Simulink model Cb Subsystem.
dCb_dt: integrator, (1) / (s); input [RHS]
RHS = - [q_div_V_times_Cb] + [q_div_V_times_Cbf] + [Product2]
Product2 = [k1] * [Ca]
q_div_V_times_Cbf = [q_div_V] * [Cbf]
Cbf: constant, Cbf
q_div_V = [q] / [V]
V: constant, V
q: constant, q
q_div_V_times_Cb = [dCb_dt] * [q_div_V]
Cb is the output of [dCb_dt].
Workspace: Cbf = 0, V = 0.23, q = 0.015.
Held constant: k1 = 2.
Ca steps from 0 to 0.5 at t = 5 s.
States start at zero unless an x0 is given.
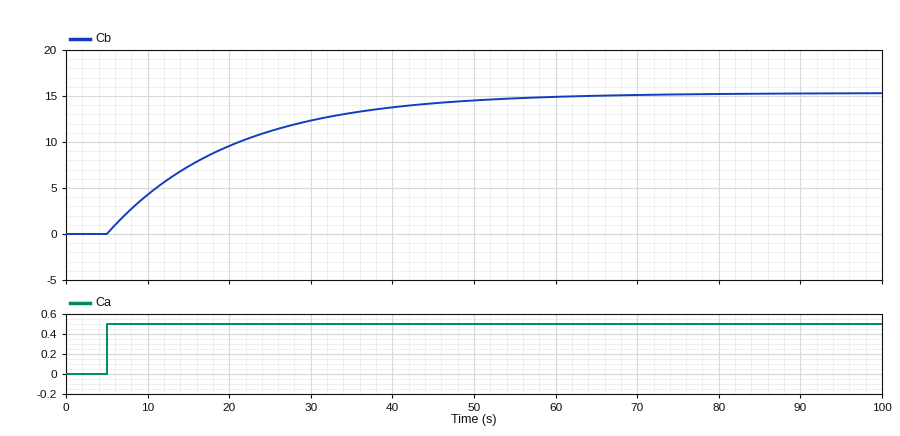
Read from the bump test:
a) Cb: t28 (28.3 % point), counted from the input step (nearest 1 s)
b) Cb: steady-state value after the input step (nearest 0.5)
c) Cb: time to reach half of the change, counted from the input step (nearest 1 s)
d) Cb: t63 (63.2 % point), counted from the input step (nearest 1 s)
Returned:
5 s
15.5
11 s
15 s
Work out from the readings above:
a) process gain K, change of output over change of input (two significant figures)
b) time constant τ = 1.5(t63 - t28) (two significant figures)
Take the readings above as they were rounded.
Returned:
31
15 s
